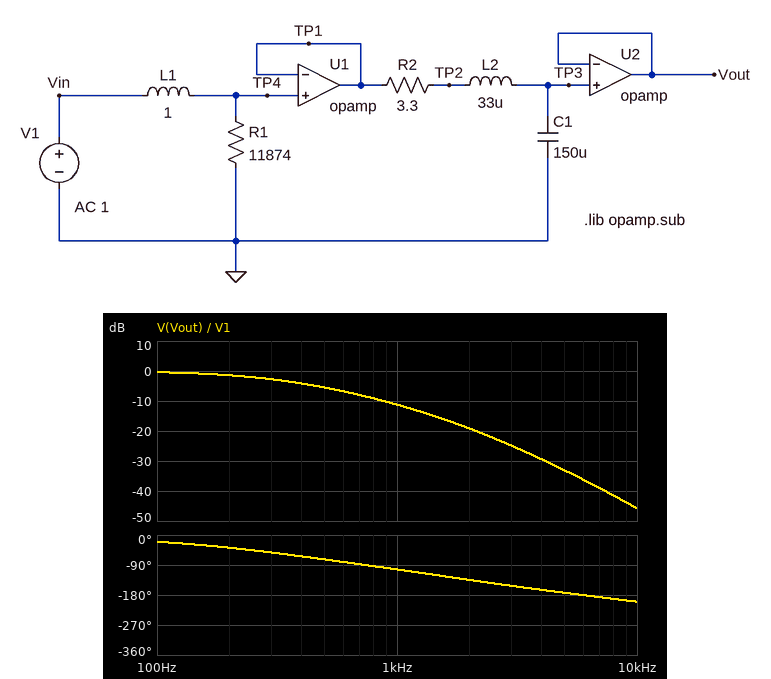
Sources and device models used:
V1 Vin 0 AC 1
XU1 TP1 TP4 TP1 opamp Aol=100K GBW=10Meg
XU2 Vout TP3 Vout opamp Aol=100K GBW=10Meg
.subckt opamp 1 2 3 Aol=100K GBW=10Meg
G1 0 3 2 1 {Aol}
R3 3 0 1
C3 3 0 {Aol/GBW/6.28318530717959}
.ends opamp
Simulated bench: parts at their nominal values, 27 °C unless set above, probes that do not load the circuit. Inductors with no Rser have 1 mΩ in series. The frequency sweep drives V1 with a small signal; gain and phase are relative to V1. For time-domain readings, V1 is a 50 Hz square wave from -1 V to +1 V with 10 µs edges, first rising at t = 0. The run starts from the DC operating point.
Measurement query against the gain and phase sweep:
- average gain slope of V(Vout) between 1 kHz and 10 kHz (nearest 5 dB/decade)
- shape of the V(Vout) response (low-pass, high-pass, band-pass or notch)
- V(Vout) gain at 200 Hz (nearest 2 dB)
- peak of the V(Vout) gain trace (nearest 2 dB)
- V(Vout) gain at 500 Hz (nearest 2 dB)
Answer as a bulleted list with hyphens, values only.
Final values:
- -35 dB/decade
- low-pass
- -2 dB
- 0 dB
- -6 dB
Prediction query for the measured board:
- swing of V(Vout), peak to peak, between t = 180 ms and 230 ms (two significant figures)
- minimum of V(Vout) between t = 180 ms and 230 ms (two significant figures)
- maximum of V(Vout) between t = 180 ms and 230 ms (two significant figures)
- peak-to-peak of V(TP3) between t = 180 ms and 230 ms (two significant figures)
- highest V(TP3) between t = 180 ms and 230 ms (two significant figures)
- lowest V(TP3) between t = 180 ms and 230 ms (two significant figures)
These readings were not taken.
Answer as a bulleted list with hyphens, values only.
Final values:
- 2.0 V
- -1.0 V
- 1.0 V
- 2.0 V
- 1.0 V
- -1.0 V
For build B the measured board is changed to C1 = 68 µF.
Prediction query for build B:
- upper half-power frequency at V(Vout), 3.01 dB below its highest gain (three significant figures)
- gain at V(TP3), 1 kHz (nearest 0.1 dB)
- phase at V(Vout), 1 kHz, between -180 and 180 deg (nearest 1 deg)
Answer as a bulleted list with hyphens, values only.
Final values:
- 657 Hz
- -5.6 dB
- -85 deg
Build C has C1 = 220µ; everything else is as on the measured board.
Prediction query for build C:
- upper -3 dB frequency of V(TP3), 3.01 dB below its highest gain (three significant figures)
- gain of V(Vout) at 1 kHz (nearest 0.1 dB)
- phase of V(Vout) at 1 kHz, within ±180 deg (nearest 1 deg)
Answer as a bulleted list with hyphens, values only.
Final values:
- 219 Hz
- -14.4 dB
- -109 deg
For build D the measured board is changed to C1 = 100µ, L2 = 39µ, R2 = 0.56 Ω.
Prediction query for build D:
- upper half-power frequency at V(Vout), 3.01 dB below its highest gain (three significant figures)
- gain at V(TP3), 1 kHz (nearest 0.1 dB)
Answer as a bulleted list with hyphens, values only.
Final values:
- 2.44 kHz
- -0.3 dB
